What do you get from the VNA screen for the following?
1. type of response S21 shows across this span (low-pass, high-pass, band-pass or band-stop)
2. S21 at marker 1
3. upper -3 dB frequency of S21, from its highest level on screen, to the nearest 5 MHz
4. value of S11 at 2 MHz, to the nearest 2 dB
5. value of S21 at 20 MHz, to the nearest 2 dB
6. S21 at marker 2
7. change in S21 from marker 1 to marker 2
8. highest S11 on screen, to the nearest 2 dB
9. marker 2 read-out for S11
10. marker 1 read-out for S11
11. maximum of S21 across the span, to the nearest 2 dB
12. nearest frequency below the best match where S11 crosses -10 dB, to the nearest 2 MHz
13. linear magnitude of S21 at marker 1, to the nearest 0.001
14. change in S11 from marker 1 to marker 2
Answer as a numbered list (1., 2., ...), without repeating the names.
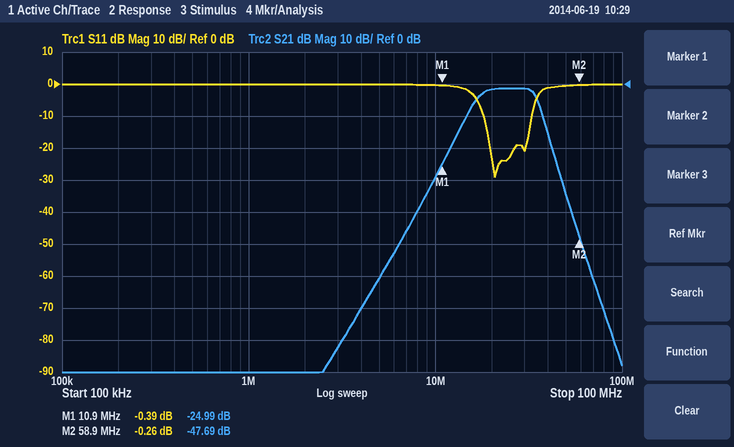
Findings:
1. band-pass
2. -24.99 dB
3. 35 MHz
4. 0 dB
5. -2 dB
6. -47.69 dB
7. -22.70 dB
8. 0 dB
9. -0.26 dB
10. -0.39 dB
11. -2 dB
12. 18 MHz
13. 0.056
14. 0.13 dB
